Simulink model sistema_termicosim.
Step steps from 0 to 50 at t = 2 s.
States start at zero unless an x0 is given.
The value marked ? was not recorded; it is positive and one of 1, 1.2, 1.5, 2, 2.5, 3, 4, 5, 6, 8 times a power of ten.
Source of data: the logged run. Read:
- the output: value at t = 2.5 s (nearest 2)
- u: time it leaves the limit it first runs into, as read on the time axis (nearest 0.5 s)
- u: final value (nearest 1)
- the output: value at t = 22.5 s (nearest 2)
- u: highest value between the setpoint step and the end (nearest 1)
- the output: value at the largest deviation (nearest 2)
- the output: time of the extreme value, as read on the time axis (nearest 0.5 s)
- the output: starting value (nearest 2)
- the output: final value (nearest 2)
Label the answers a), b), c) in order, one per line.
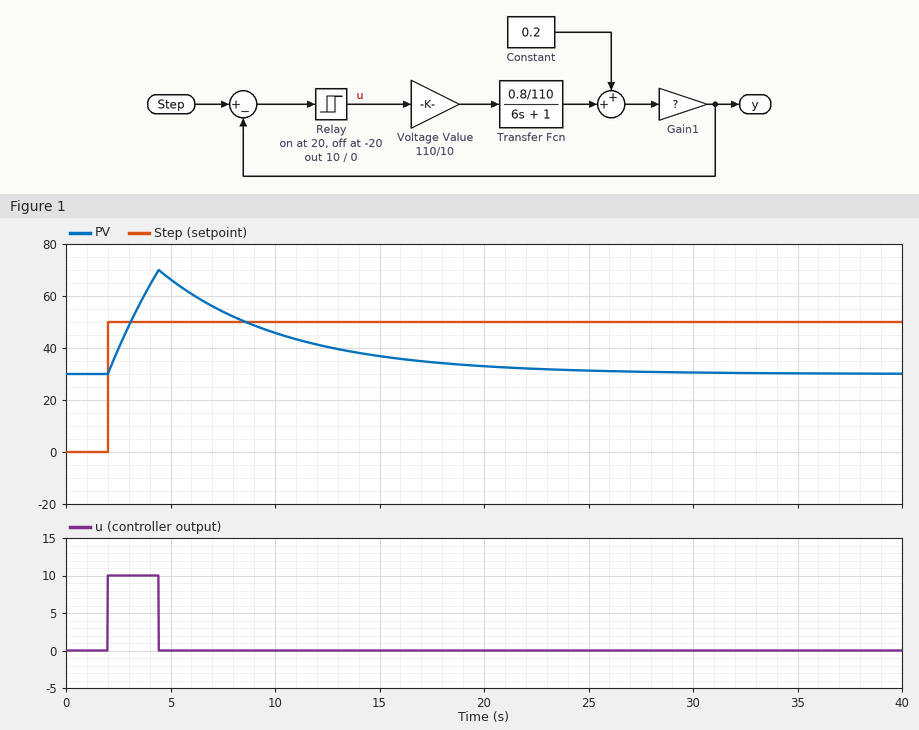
a) 40
b) 4.5 s
c) 0
d) 32
e) 10
f) 70
g) 4.5 s
h) 30
i) 30
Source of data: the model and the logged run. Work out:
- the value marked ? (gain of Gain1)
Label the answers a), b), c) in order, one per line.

a) 150
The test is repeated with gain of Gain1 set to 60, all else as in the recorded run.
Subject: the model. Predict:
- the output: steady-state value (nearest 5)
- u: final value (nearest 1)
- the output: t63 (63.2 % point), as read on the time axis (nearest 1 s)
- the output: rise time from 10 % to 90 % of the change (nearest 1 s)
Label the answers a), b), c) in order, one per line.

a) 60
b) 10
c) 8 s
d) 13 s
